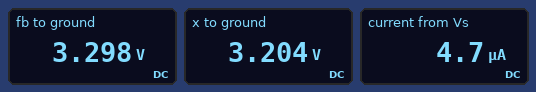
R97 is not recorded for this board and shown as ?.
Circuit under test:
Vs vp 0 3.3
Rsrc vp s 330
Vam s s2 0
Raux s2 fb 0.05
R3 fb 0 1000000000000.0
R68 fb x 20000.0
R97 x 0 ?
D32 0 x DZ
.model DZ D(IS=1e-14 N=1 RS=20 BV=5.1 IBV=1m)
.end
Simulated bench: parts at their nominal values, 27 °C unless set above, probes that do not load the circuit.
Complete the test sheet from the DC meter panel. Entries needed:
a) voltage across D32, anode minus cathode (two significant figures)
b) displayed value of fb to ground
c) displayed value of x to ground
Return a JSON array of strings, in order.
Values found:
["-3.2 V", "3.298 V", "3.204 V"]
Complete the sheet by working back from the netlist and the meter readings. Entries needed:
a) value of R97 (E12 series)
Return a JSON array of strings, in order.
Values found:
["680 kΩ"]
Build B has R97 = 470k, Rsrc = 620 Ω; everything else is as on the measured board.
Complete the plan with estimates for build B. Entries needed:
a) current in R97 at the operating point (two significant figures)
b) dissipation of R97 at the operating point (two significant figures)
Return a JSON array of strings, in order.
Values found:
["6.7 µA", "21 µW"]
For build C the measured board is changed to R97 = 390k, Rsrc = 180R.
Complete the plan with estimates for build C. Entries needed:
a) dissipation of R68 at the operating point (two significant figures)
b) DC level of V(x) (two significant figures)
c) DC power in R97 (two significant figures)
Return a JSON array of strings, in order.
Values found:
["1.3 µW", "3.1 V", "25 µW"]
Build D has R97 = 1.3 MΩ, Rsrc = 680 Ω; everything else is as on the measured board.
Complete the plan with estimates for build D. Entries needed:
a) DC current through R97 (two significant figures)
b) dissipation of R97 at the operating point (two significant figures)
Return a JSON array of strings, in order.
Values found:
["2.5 µA", "8.1 µW"]
